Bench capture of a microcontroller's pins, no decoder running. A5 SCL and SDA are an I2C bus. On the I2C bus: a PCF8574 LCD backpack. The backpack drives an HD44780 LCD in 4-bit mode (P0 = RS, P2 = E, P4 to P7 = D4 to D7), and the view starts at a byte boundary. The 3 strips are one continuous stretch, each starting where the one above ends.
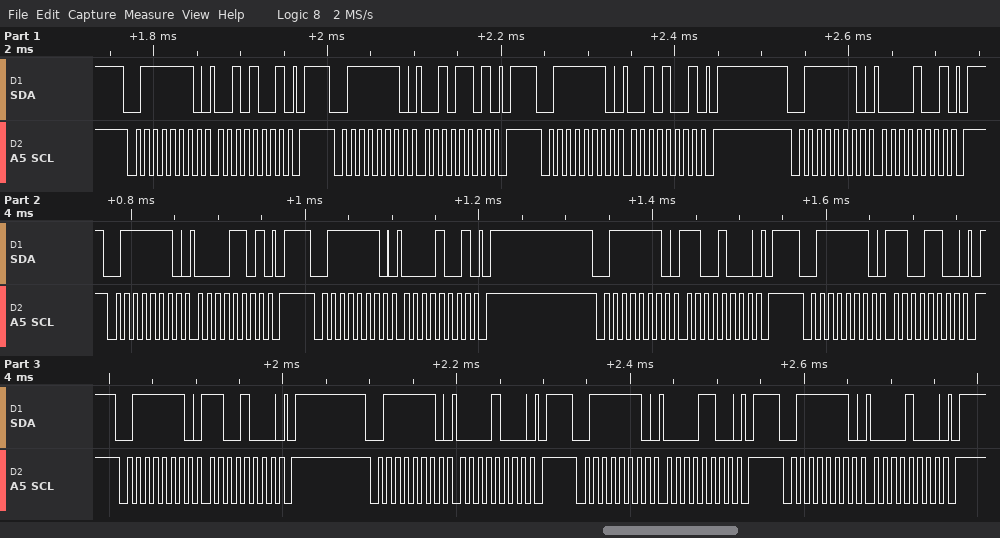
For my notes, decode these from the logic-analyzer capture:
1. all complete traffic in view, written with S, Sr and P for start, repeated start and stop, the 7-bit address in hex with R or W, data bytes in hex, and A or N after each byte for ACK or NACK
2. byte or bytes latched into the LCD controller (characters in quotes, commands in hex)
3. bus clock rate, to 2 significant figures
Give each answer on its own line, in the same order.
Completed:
S 3FW A 29 A P S 3FW A 2D A P S 3FW A 29 A P S 3FW A 09 A P S 3FW A 0D A P S 3FW A 09 A P S 3FW A C8 A P S 3FW A CC A P S 3FW A C8 A P S 3FW A 08 A P S 3FW A 0C A P S 3FW A 08 A P
' ' 0xC0
100 kHz
